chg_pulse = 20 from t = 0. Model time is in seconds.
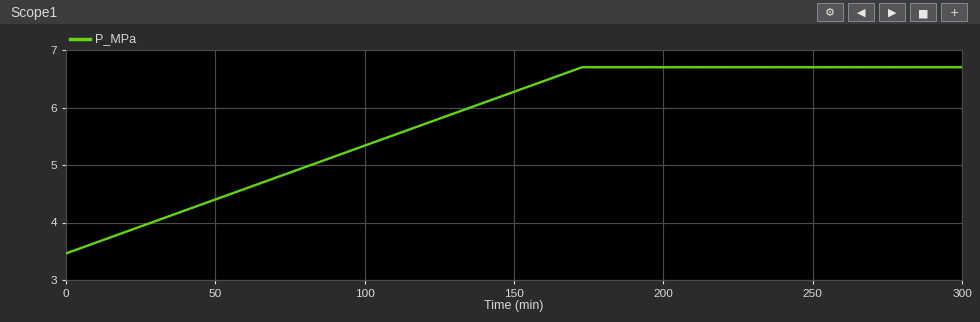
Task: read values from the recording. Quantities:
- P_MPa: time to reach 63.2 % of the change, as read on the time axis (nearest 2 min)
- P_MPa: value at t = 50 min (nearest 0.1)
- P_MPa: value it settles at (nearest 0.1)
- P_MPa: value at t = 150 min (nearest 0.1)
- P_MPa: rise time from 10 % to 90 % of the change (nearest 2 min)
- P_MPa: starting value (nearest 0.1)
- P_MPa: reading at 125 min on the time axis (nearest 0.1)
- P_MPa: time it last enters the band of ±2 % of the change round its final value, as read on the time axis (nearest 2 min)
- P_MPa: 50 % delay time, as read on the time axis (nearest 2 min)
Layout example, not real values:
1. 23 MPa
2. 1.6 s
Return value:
1. 110 min
2. 4.4
3. 6.7
4. 6.3
5. 138 min
6. 3.5
7. 5.8
8. 170 min
9. 86 min
